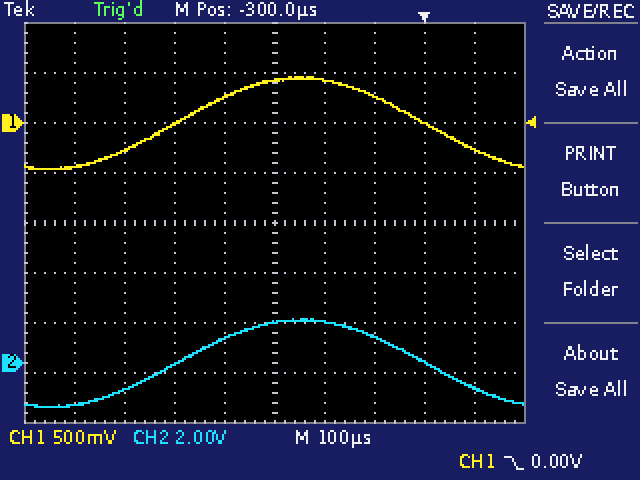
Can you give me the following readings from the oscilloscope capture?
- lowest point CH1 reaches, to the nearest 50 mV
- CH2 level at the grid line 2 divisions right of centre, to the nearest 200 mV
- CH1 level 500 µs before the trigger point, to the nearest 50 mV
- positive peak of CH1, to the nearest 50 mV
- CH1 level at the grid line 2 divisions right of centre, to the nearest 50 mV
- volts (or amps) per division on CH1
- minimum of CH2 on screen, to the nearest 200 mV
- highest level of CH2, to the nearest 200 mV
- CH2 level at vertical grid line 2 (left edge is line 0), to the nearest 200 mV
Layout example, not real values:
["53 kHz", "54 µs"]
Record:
["-450 mV", "1.0 V", "0 mV", "450 mV", "250 mV", "500 mV", "-1.8 V", "1.8 V", "-1.0 V"]
